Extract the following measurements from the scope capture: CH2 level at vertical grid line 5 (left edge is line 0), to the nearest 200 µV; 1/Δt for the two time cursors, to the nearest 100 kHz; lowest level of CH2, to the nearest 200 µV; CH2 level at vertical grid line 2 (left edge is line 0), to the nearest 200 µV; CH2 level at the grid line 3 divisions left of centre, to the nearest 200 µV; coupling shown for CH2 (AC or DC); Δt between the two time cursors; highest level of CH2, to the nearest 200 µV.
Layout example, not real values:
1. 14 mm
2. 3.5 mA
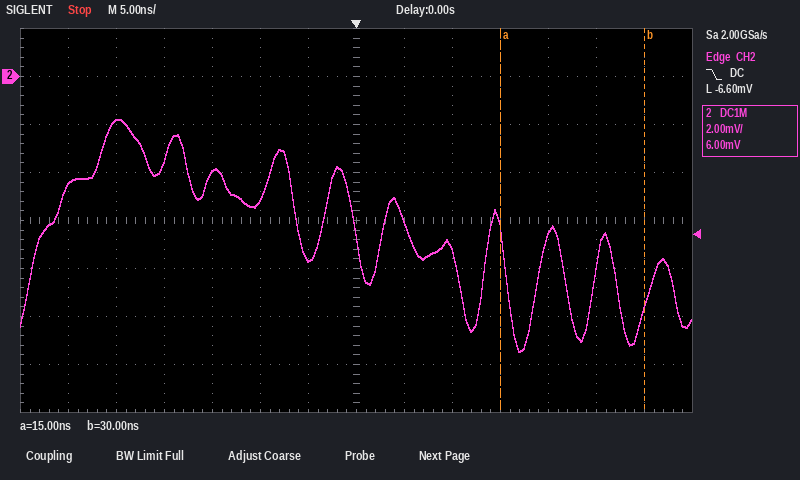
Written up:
1. -5.2 mV
2. 66.7 MHz
3. -11.4 mV
4. -1.8 mV
5. -4.0 mV
6. DC
7. 15.0 ns
8. -1.8 mV
